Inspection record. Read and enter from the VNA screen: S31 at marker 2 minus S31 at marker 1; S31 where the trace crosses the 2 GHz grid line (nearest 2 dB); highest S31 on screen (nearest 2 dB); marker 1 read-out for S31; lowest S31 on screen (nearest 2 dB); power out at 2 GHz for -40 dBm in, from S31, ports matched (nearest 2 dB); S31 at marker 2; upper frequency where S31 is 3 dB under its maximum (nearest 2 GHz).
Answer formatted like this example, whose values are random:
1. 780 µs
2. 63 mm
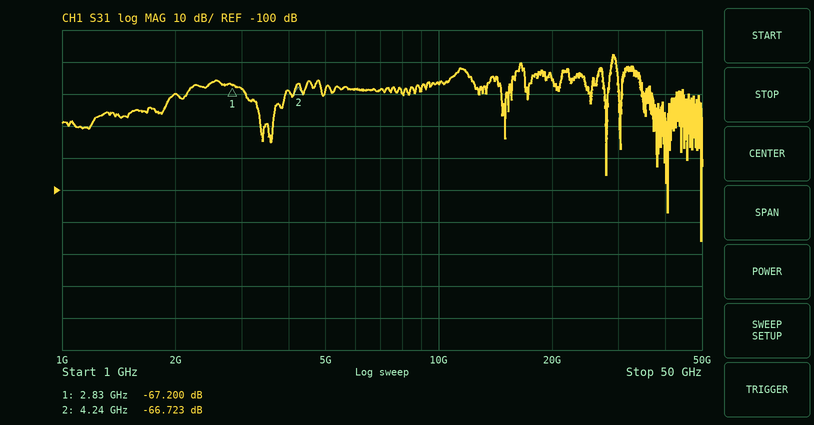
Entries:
1. 0.477 dB
2. -70 dB
3. -58 dB
4. -67.200 dB
5. -116 dB
6. -110 dBm
7. -66.723 dB
8. 30 GHz
